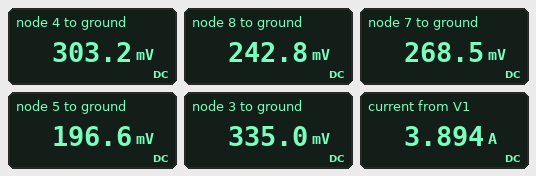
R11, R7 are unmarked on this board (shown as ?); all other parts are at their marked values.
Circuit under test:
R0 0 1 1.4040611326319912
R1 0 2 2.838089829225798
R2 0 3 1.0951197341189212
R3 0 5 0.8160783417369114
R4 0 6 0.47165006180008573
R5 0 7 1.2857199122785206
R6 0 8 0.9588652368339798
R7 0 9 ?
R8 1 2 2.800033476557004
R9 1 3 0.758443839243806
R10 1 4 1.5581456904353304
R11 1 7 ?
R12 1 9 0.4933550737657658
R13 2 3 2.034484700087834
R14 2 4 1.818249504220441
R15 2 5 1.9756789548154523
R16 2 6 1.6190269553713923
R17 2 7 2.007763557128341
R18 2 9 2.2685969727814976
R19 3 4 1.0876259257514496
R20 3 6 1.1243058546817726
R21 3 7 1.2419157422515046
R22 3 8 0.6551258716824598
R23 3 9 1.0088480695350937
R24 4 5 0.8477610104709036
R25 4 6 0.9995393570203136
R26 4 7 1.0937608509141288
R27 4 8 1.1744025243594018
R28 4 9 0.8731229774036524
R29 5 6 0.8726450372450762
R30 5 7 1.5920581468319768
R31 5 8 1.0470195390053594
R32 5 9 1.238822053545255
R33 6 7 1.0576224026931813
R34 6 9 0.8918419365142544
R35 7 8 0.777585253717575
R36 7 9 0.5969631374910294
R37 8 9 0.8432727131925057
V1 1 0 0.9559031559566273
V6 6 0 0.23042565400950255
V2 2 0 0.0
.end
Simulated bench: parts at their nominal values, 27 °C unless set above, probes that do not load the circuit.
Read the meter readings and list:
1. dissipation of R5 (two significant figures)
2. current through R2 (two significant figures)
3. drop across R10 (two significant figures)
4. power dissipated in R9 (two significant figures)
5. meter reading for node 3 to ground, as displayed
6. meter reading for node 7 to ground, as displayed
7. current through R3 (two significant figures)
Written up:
56 mW
310 mA
650 mV
510 mW
335.0 mV
268.5 mV
240 mA
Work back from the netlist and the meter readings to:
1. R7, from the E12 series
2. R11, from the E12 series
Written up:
0.33 Ω
2.2 Ω
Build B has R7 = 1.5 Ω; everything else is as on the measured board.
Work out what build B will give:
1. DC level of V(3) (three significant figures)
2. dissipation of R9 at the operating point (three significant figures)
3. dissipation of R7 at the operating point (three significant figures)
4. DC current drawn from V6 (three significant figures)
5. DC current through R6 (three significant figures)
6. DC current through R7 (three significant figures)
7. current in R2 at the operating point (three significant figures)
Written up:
359 mV
469 mW
102 mW
178 mA
288 mA
261 mA
328 mA
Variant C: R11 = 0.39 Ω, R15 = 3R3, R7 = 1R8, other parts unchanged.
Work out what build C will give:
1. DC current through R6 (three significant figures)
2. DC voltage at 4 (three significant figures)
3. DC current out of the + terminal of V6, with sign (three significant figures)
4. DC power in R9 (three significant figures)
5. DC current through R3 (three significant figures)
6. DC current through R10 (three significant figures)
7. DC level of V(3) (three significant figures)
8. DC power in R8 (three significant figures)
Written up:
354 mA
383 mV
-183 mA
406 mW
332 mA
368 mA
401 mV
326 mW
